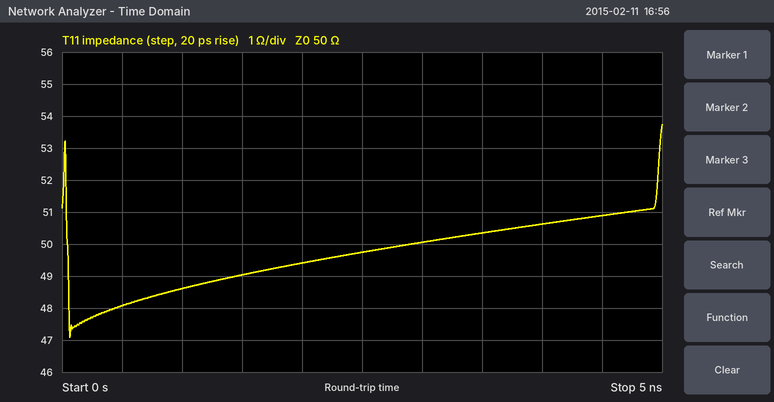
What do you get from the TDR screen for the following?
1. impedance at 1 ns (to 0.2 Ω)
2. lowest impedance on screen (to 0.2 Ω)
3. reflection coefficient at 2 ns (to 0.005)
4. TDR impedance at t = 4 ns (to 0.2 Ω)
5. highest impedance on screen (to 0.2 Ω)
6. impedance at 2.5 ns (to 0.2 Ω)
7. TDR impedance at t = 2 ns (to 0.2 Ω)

48.6 Ω
47.0 Ω
-0.005
50.6 Ω
53.8 Ω
49.8 Ω
49.4 Ω
